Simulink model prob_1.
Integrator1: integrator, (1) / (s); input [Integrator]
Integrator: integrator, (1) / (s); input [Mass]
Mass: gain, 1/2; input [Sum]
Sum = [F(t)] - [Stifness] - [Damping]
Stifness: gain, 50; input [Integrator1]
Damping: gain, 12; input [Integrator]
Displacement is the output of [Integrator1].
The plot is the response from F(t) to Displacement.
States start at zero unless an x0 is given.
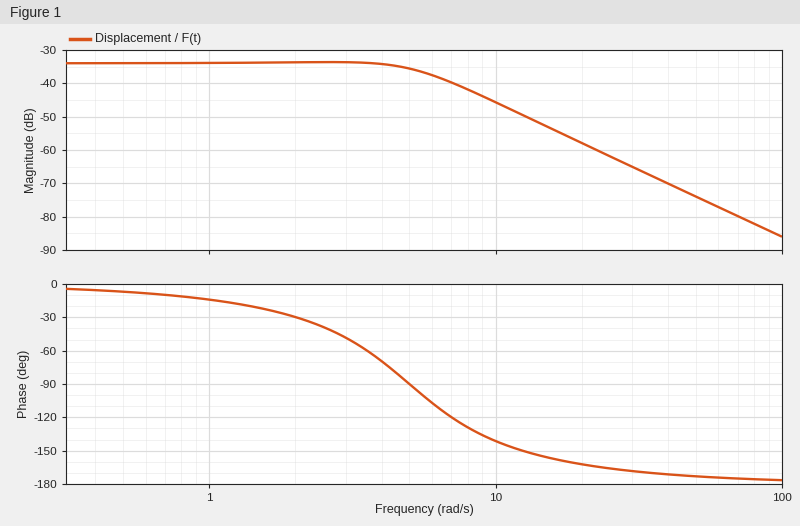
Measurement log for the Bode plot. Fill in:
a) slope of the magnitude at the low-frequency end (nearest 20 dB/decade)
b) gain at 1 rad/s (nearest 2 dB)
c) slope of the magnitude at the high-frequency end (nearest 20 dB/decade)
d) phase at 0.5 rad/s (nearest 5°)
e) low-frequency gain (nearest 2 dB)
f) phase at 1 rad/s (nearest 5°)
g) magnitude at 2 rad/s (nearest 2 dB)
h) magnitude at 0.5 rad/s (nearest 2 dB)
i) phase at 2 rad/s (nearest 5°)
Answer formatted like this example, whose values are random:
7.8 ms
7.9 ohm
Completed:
0 dB/decade
-34 dB
-40 dB/decade
-5°
-34 dB
-15°
-34 dB
-34 dB
-30°
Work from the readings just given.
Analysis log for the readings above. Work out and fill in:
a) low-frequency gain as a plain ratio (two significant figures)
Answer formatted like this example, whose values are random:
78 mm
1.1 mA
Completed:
0.020
